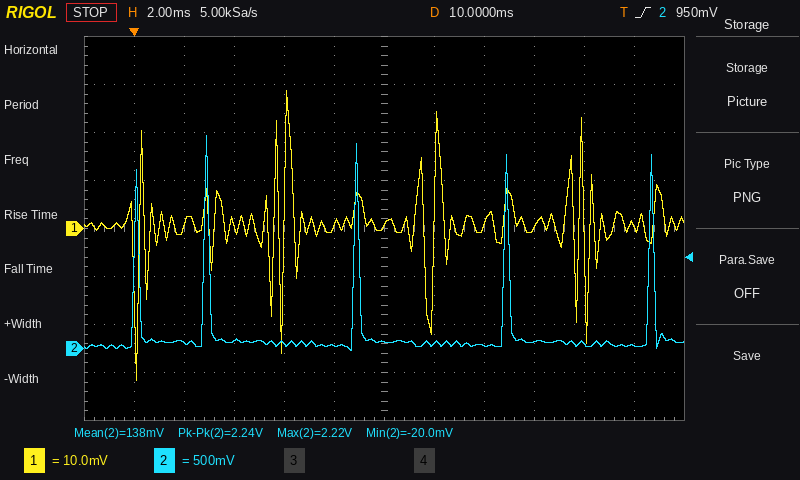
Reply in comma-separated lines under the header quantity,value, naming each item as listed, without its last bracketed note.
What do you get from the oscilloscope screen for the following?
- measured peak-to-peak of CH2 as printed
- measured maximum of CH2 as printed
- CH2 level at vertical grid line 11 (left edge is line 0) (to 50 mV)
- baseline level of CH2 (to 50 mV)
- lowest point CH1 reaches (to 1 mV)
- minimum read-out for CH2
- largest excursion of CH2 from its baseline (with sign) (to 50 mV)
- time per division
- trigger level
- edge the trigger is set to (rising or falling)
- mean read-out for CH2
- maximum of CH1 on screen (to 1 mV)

quantity,value
measured peak-to-peak of CH2 as printed,2.24 V
measured maximum of CH2 as printed,2.22 V
CH2 level at vertical grid line 11 (left edge is line 0),50 mV
baseline level of CH2,50 mV
lowest point CH1 reaches,-32 mV
minimum read-out for CH2,-20.0 mV
largest excursion of CH2 from its baseline (with sign),+2.15 V
time per division,2 ms
trigger level,950 mV
edge the trigger is set to,rising
mean read-out for CH2,138 mV
maximum of CH1 on screen,29 mV
